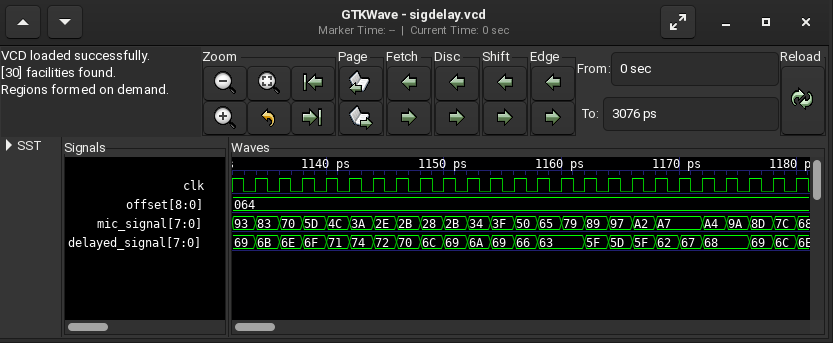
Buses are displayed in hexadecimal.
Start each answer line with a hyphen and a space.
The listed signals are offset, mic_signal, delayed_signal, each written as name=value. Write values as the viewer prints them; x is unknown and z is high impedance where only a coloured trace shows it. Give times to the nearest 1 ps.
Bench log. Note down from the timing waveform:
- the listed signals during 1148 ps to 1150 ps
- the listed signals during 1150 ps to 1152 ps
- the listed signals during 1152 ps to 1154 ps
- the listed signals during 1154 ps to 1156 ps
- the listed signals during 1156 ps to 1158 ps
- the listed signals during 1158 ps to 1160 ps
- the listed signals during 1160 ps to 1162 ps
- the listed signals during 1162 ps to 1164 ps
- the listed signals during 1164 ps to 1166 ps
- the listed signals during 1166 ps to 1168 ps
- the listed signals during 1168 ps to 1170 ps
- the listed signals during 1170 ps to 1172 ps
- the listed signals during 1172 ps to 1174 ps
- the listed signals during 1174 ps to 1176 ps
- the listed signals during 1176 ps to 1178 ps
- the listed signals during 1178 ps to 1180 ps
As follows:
- offset=064, mic_signal=28, delayed_signal=6C
- offset=064, mic_signal=2B, delayed_signal=69
- offset=064, mic_signal=34, delayed_signal=6A
- offset=064, mic_signal=3F, delayed_signal=69
- offset=064, mic_signal=50, delayed_signal=66
- offset=064, mic_signal=65, delayed_signal=63
- offset=064, mic_signal=79, delayed_signal=63
- offset=064, mic_signal=89, delayed_signal=5F
- offset=064, mic_signal=97, delayed_signal=5D
- offset=064, mic_signal=A2, delayed_signal=5F
- offset=064, mic_signal=A7, delayed_signal=62
- offset=064, mic_signal=A7, delayed_signal=67
- offset=064, mic_signal=A4, delayed_signal=68
- offset=064, mic_signal=9A, delayed_signal=68
- offset=064, mic_signal=8D, delayed_signal=69
- offset=064, mic_signal=7C, delayed_signal=6C
